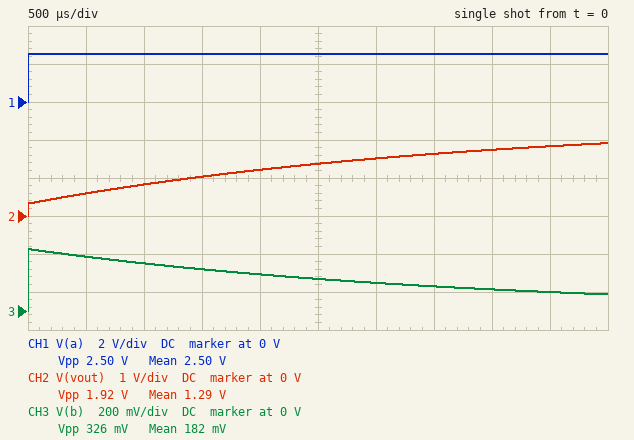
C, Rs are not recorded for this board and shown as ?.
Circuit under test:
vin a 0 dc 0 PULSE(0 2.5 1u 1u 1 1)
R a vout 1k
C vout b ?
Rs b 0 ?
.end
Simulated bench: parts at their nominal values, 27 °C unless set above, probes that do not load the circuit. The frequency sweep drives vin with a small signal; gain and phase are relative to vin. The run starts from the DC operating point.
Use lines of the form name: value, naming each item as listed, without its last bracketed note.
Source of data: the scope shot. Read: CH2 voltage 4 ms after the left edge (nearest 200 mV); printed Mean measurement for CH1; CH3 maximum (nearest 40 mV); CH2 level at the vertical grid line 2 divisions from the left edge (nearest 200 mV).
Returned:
CH2 voltage 4 ms after the left edge: 1.8 V
printed Mean measurement for CH1: 2.50 V
CH3 maximum: 320 mV
CH2 level at the vertical grid line 2 divisions from the left edge: 800 mV
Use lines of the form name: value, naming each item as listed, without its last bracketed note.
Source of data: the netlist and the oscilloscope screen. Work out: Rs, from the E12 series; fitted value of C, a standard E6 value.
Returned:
Rs, from the E12 series: 150 Ω
fitted value of C, a standard E6 value: 3.3 µF
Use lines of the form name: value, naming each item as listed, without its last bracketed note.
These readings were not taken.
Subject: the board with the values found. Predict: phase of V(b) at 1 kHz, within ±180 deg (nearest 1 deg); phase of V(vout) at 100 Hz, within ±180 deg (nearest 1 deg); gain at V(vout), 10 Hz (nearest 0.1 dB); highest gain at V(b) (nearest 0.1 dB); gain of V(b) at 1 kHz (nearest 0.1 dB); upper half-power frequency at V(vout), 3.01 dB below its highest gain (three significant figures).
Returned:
phase of V(b) at 1 kHz, within ±180 deg: 2 deg
phase of V(vout) at 100 Hz, within ±180 deg: -50 deg
gain at V(vout), 10 Hz: -0.2 dB
highest gain at V(b): -17.7 dB
gain of V(b) at 1 kHz: -17.7 dB
upper half-power frequency at V(vout), 3.01 dB below its highest gain: 42.7 Hz
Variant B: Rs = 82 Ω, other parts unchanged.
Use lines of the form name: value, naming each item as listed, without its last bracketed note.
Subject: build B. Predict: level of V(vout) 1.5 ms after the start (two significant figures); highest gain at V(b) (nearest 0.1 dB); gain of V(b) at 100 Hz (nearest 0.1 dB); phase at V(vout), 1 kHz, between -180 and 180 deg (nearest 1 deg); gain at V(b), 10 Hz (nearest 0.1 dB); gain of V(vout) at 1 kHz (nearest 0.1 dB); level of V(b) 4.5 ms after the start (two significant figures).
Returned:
level of V(vout) 1.5 ms after the start: 980 mV
highest gain at V(b): -22.4 dB
gain of V(b) at 100 Hz: -23.2 dB
phase at V(vout), 1 kHz, between -180 and 180 deg: -28 deg
gain at V(b), 10 Hz: -35.6 dB
gain of V(vout) at 1 kHz: -21.1 dB
level of V(b) 4.5 ms after the start: 54 mV
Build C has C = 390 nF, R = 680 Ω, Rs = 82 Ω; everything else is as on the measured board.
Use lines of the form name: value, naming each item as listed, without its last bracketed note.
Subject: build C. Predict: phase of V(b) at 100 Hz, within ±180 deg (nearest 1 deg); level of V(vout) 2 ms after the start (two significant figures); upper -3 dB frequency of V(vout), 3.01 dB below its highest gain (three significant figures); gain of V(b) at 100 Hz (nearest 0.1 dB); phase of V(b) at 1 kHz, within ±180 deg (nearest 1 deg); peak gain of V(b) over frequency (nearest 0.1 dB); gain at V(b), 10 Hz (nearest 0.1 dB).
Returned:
phase of V(b) at 100 Hz, within ±180 deg: 79 deg
level of V(vout) 2 ms after the start: 2.5 V
upper -3 dB frequency of V(vout), 3.01 dB below its highest gain: 542 Hz
gain of V(b) at 100 Hz: -34.1 dB
phase of V(b) at 1 kHz, within ±180 deg: 28 deg
peak gain of V(b) over frequency: -19.4 dB
gain at V(b), 10 Hz: -53.9 dB
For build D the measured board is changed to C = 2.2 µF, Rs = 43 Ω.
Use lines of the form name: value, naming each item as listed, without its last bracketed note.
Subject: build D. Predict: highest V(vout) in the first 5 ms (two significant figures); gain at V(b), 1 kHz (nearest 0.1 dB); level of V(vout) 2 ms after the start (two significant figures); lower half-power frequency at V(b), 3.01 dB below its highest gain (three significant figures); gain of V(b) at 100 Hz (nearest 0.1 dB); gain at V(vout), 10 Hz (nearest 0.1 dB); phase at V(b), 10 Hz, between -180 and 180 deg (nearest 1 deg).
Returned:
highest V(vout) in the first 5 ms: 2.2 V
gain at V(b), 1 kHz: -27.7 dB
level of V(vout) 2 ms after the start: 1.5 V
lower half-power frequency at V(b), 3.01 dB below its highest gain: 69.4 Hz
gain of V(b) at 100 Hz: -29.4 dB
gain at V(vout), 10 Hz: -0.1 dB
phase at V(b), 10 Hz, between -180 and 180 deg: 82 deg
